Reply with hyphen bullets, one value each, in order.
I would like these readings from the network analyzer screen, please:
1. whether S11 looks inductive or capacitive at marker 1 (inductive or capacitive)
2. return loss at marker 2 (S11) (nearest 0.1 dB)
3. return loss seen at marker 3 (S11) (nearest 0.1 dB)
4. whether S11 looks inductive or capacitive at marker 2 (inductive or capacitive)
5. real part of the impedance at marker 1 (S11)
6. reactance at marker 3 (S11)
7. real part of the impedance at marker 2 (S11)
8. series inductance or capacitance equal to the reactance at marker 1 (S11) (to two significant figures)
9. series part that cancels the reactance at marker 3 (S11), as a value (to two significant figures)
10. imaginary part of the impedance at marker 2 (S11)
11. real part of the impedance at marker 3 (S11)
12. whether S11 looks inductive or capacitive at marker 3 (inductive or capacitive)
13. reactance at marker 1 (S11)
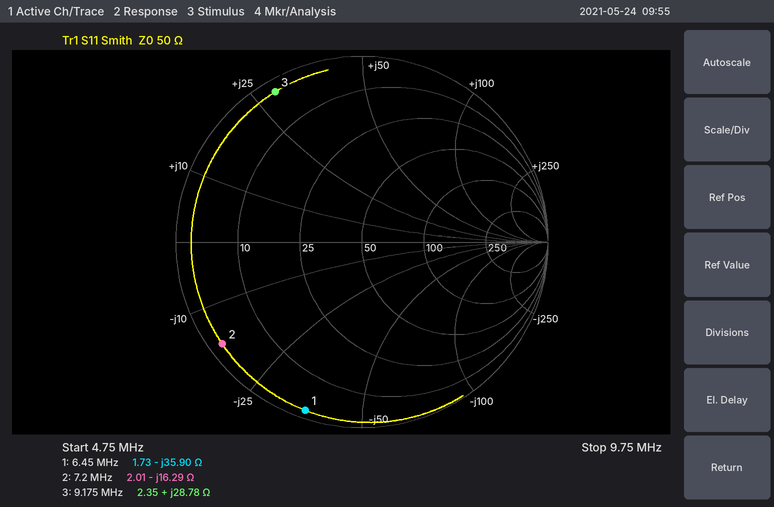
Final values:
- capacitive
- 0.6 dB
- 0.6 dB
- capacitive
- 1.73 Ω
- +28.78 Ω
- 2.01 Ω
- 690 pF
- 600 pF
- -16.29 Ω
- 2.35 Ω
- inductive
- -35.90 Ω
